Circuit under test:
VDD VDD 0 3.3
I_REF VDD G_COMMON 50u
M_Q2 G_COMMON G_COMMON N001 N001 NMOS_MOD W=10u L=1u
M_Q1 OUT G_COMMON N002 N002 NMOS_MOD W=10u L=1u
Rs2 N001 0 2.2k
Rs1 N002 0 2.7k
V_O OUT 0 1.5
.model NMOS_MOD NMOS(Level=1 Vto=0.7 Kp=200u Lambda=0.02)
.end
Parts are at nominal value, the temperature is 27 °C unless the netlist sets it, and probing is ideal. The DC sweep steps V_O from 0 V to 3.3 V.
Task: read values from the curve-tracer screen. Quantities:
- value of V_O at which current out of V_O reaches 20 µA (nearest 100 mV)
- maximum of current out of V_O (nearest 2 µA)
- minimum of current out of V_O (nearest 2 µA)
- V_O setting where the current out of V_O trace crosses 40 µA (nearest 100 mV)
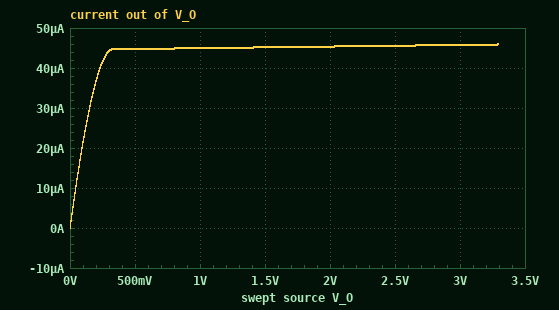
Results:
100 mV
46 µA
0 A
200 mV
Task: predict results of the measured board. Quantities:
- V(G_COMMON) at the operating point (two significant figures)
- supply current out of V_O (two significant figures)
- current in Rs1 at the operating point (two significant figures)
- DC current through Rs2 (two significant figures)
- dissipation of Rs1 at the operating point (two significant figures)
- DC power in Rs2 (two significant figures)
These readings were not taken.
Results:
1.0 V
45 µA
45 µA
50 µA
5.5 µW
5.5 µW
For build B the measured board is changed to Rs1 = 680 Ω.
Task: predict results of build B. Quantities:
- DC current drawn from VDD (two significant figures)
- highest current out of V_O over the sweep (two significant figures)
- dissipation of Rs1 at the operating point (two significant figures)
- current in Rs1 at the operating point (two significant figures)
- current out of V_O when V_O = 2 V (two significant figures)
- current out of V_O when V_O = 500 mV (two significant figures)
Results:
50 µA
81 µA
4.3 µW
79 µA
80 µA
78 µA
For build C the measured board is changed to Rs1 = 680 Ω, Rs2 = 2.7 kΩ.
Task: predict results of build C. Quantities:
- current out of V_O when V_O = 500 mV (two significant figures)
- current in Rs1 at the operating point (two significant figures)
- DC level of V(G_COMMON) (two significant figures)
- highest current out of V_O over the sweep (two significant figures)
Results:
89 µA
90 µA
1.1 V
92 µA
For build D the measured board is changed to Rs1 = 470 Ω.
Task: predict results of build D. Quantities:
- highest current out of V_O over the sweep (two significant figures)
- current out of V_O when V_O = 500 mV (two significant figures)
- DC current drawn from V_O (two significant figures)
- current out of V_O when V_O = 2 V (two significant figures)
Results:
89 µA
86 µA
87 µA
88 µA
